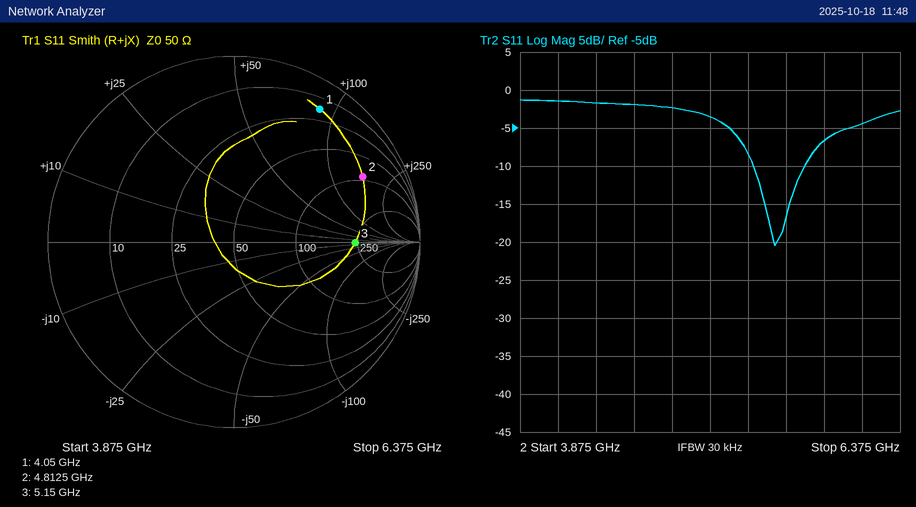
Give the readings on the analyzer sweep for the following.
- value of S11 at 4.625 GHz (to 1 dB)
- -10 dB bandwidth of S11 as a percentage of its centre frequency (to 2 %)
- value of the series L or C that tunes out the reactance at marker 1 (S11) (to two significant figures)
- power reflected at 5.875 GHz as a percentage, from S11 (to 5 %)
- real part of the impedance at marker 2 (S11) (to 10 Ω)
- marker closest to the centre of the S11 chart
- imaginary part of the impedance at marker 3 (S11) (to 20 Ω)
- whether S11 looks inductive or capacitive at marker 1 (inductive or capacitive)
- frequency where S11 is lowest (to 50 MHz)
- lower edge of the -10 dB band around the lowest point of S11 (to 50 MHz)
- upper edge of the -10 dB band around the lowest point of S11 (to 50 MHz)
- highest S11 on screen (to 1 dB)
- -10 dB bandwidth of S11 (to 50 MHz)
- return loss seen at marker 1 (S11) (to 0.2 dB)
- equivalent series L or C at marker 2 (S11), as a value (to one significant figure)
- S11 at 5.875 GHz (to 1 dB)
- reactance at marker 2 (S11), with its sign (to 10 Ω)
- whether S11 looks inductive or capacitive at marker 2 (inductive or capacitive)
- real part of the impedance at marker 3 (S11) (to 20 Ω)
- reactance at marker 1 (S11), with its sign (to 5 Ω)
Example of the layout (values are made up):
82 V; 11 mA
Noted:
-2 dB; 6 %; 440 fF; 20 %; 90 Ω; marker 3; 0 Ω; inductive; 5.55 GHz; 5.40 GHz; 5.75 GHz; -1 dB; 350 MHz; 1.4 dB; 5 nH; -7 dB; +160 Ω; inductive; 240 Ω; +90 Ω
